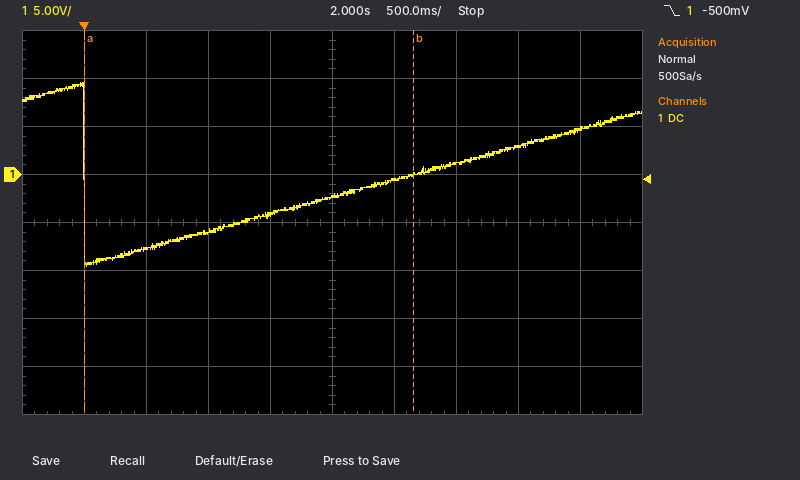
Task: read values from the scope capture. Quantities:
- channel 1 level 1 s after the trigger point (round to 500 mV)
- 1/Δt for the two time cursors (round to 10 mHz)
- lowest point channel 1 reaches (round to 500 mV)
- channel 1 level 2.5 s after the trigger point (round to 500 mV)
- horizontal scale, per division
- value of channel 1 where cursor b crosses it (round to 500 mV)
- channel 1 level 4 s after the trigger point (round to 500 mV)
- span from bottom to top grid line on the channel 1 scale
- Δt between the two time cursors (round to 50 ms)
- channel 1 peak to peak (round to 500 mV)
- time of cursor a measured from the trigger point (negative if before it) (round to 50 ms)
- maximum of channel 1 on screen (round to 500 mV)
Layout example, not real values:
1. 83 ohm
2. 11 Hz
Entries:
1. -6.0 V
2. 380 mHz
3. -9.5 V
4. -500 mV
5. 500 ms
6. 0.0 V
7. 4.5 V
8. 40 V
9. 2.65 s
10. 19.0 V
11. 0 ms
12. 9.5 V
